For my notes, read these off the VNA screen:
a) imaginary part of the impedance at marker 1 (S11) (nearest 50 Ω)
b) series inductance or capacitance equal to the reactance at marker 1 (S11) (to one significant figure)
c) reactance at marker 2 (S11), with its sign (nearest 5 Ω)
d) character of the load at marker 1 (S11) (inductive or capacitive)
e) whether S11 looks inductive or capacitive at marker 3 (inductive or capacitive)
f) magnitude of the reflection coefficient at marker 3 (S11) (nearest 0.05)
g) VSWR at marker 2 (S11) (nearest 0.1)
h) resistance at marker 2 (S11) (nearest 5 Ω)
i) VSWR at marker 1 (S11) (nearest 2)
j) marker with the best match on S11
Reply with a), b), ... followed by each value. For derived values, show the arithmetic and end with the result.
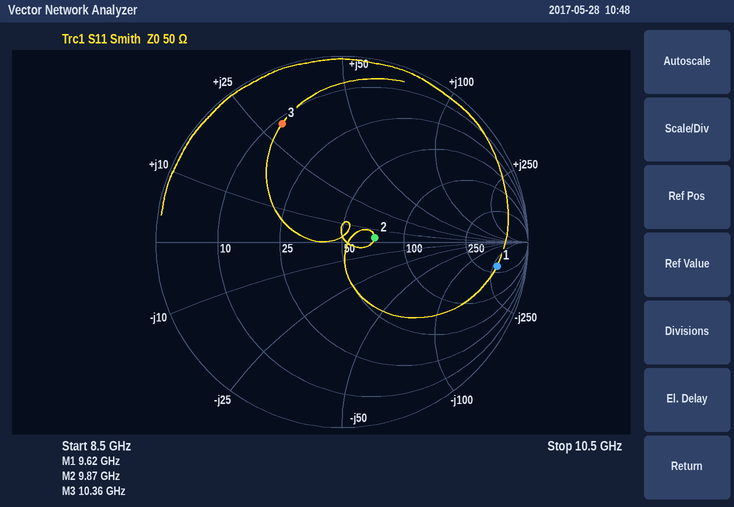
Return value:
a) -300 Ω
b) C = 1/(2π × 9.62 GHz × 300 Ω) ≈ 55.1 fF, so 60 fF to one significant figure
c) +5 Ω
d) capacitive
e) inductive
f) 0.70
g) 1.4
h) 70 Ω
i) 12
j) marker 2
